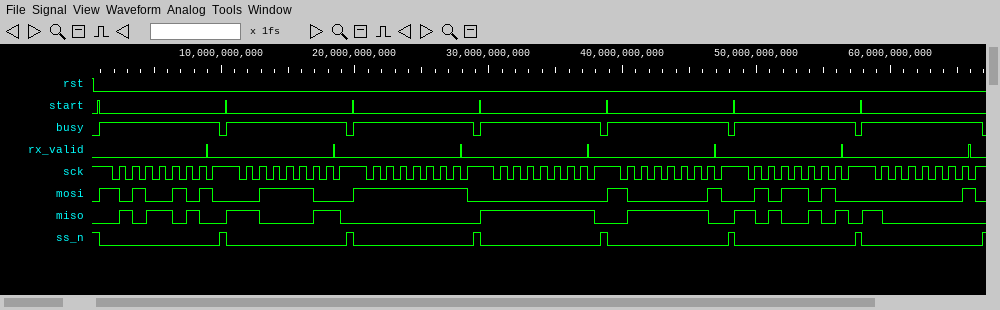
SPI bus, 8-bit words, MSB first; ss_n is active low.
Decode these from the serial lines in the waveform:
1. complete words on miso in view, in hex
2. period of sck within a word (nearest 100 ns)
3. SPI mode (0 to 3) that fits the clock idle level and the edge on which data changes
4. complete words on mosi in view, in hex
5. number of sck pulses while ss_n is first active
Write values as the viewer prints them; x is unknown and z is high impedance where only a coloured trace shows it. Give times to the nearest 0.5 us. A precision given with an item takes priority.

5A, C3, 00, FF, 7E, A5, 80
1000 ns
2
A5, 3C, FF, 00, 81, 5A, 01
8
